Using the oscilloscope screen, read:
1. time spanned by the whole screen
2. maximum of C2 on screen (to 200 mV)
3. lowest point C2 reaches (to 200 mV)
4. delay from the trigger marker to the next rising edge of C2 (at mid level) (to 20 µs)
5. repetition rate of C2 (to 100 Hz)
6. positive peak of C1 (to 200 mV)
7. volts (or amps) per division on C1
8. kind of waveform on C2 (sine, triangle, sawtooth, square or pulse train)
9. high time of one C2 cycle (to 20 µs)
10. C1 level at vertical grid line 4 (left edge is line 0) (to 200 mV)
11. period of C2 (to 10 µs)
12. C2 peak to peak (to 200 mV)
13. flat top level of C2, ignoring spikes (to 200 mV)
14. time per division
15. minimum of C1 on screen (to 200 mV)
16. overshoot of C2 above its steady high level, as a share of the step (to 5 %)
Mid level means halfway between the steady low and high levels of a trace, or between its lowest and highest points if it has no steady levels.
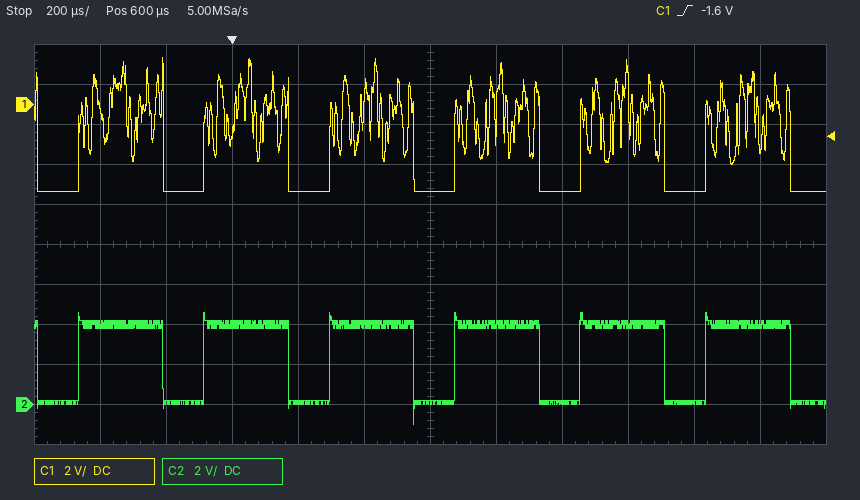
2.4 ms
4.6 V
-1.0 V
300 µs
2.6 kHz
2.4 V
2 V
pulse train
260 µs
-4.4 V
380 µs
5.6 V
4.0 V
200 µs
-4.4 V
15 %
